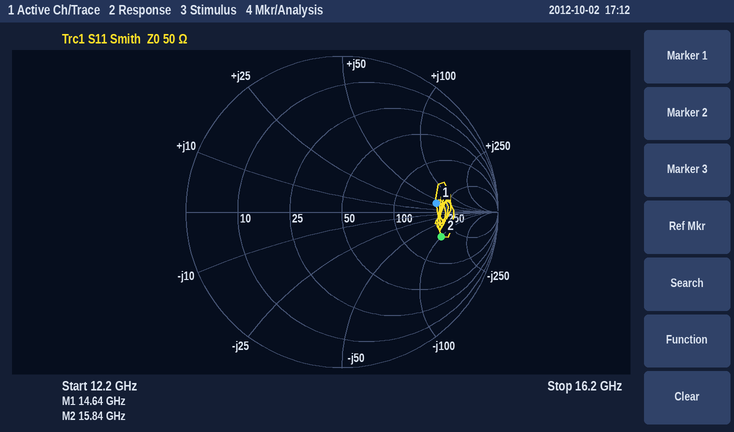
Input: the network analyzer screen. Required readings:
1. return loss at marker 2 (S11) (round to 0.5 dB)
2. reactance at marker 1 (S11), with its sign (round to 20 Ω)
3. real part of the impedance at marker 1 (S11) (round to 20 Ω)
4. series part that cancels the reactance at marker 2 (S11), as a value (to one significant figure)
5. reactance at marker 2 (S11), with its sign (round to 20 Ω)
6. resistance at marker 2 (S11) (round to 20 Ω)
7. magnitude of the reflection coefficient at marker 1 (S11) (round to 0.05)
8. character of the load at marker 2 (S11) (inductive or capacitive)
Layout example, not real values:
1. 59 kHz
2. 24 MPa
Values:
1. 3.5 dB
2. +40 Ω
3. 200 Ω
4. 1 nH
5. -100 Ω
6. 180 Ω
7. 0.60
8. capacitive
